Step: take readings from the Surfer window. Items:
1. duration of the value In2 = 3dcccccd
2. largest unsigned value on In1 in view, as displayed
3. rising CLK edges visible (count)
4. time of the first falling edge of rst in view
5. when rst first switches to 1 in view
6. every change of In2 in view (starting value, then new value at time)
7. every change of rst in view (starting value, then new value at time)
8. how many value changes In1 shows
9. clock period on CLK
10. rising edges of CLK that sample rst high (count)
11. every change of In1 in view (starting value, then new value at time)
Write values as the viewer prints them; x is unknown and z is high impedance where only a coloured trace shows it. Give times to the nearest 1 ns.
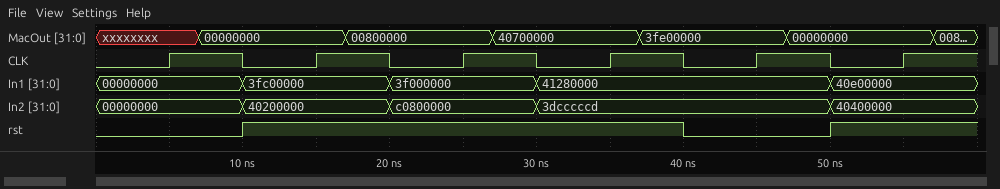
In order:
20 ns
41280000
6
40 ns
10 ns
00000000, 40200000 at 10 ns, c0800000 at 20 ns, 3dcccccd at 30 ns, 40400000 at 50 ns
0, 1 at 10 ns, 0 at 40 ns, 1 at 50 ns
4
10 ns
4
00000000, 3fc00000 at 10 ns, 3f000000 at 20 ns, 41280000 at 30 ns, 40e00000 at 50 ns
